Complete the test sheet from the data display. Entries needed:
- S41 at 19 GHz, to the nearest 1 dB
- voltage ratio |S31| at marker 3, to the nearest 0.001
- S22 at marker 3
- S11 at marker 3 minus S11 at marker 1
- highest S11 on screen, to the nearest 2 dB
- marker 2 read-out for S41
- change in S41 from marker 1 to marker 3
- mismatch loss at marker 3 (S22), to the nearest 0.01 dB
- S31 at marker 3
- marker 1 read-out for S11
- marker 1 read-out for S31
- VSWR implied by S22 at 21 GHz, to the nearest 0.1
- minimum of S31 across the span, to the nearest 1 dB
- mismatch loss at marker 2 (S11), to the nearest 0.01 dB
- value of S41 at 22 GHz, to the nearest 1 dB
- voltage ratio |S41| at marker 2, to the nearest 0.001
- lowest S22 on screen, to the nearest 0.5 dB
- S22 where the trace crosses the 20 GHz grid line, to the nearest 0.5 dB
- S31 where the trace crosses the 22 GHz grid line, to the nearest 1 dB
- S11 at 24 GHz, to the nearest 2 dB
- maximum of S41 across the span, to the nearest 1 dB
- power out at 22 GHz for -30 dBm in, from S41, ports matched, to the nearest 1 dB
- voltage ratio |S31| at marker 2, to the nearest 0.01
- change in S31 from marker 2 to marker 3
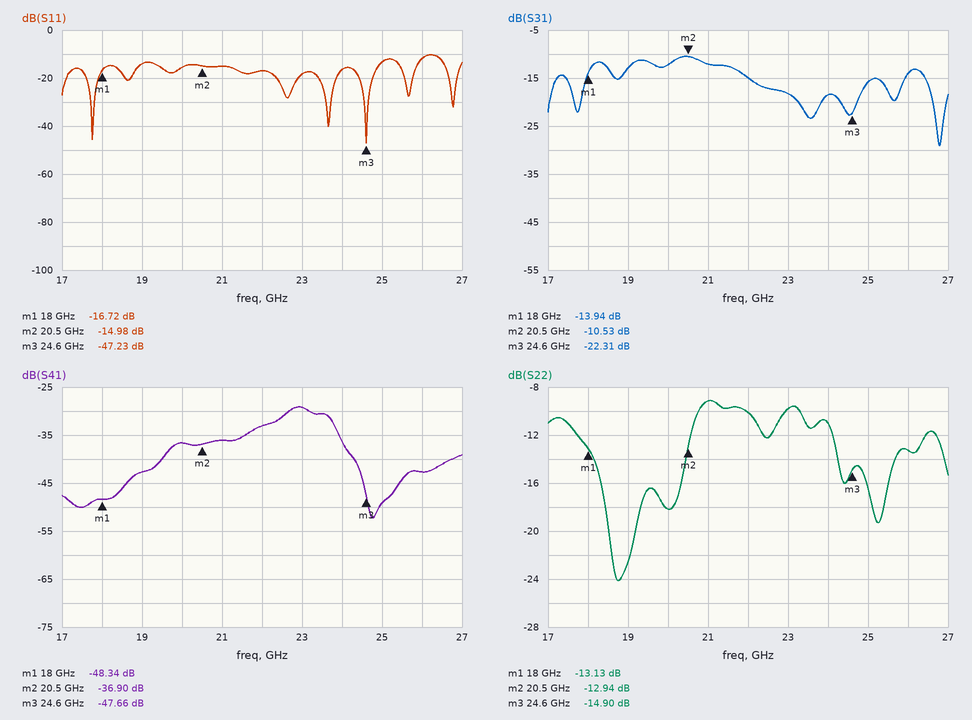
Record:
-43 dB
0.077
-14.90 dB
-30.51 dB
-10 dB
-36.90 dB
0.68 dB
0.14 dB
-22.31 dB
-16.72 dB
-13.94 dB
2.1
-29 dB
0.14 dB
-33 dB
0.014
-24.0 dB
-18.0 dB
-15 dB
-16 dB
-29 dB
-63 dBm
0.30
-11.78 dB
